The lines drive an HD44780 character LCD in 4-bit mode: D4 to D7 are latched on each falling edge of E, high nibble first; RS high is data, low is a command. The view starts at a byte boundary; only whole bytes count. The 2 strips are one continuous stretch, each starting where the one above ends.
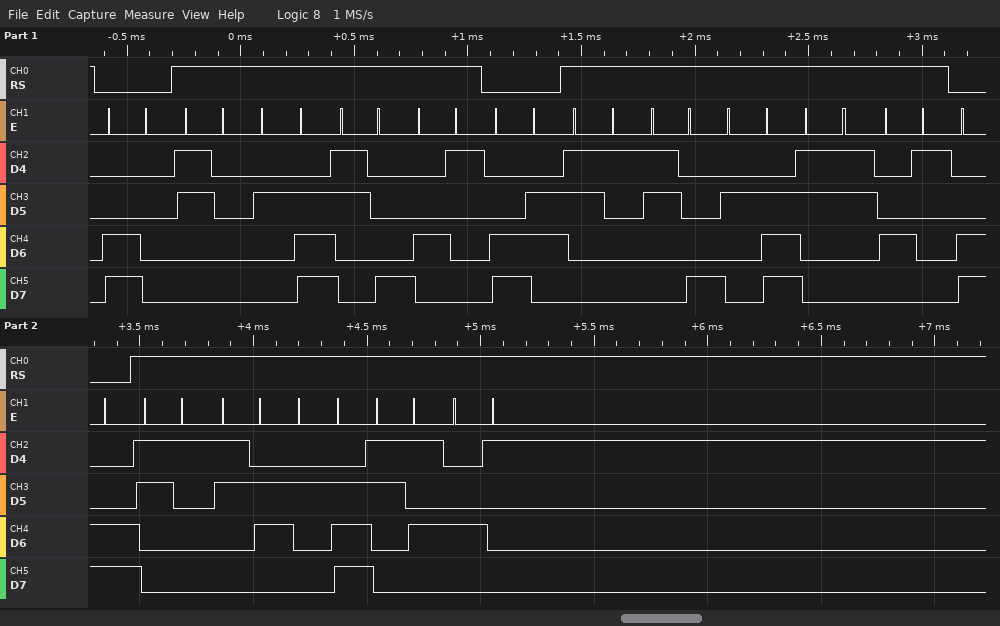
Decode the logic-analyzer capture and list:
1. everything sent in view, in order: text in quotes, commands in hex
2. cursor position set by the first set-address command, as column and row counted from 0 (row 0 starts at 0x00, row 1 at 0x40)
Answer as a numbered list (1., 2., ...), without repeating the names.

1. 0xC0 "0.8A" 0xC6 "18.3A" 0xCC "16.5A"
2. column 0, row 1
